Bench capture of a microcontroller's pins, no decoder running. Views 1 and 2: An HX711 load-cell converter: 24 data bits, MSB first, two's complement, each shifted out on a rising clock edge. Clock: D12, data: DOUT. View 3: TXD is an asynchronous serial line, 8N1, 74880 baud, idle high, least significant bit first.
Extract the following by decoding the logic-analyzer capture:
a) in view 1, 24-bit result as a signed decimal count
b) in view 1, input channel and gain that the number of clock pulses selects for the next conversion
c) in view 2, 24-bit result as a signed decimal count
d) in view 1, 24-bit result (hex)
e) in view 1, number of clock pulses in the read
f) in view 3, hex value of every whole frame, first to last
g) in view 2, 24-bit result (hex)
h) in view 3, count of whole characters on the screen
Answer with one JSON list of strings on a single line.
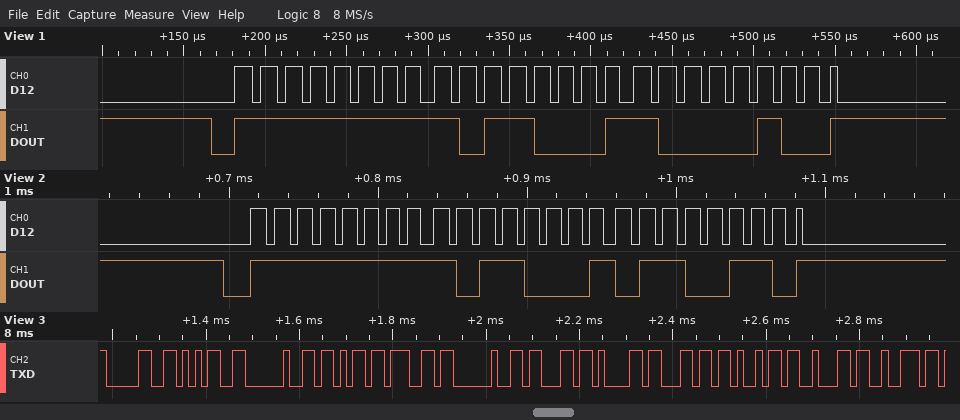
["-20092", "channel A, gain 128", "-20122", "0xFFB184", "25", "30 35 20 6B 67 20 63 61 6C 69 62 72", "0xFFB166", "12"]
